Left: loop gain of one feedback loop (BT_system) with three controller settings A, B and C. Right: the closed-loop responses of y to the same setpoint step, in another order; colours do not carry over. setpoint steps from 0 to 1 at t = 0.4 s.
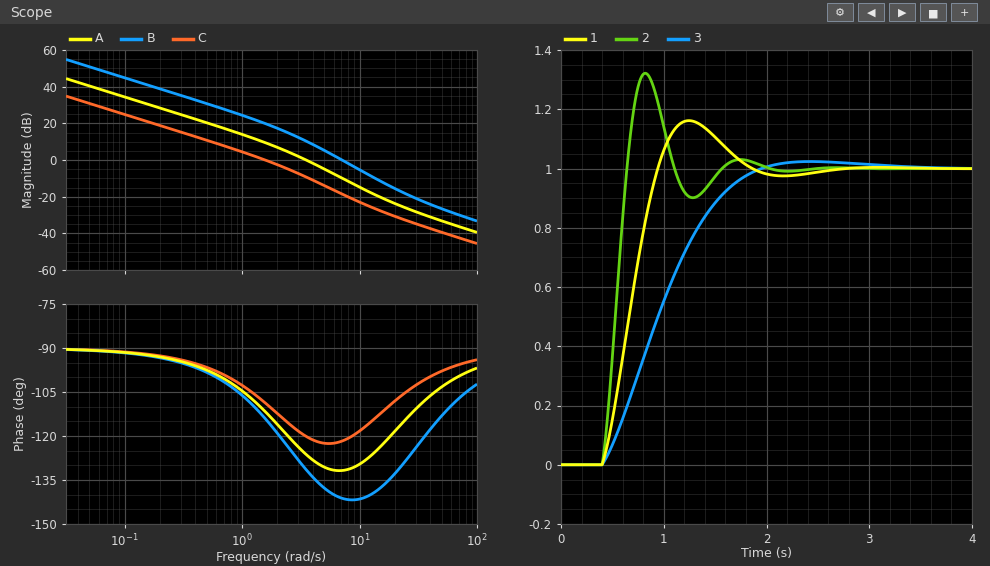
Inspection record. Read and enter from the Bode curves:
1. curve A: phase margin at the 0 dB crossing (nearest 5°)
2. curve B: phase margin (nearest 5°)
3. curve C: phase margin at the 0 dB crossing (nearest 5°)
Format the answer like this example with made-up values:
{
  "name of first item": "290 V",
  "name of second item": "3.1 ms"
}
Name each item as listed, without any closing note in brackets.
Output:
{
  "curve A: phase margin at the 0 dB crossing": "55°",
  "curve B: phase margin": "40°",
  "curve C: phase margin at the 0 dB crossing": "70°"
}
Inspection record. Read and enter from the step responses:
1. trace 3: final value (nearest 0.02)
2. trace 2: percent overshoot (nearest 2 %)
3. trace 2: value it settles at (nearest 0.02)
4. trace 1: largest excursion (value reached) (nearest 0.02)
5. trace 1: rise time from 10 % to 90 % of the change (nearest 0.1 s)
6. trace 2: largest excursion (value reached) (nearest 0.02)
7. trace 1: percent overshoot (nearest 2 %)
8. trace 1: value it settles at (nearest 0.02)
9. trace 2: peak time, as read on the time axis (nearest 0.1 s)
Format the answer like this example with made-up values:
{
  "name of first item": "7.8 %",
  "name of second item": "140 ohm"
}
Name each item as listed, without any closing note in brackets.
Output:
{
  "trace 3: final value": "1.00",
  "trace 2: percent overshoot": "32 %",
  "trace 2: value it settles at": "1.00",
  "trace 1: largest excursion (value reached)": "1.16",
  "trace 1: rise time from 10 % to 90 % of the change": "0.4 s",
  "trace 2: largest excursion (value reached)": "1.32",
  "trace 1: percent overshoot": "16 %",
  "trace 1: value it settles at": "1.00",
  "trace 2: peak time, as read on the time axis": "0.8 s"
}
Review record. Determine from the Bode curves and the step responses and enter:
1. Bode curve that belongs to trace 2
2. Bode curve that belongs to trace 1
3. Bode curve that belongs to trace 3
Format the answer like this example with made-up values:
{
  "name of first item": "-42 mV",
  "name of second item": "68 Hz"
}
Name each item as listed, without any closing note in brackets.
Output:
{
  "Bode curve that belongs to trace 2": "B",
  "Bode curve that belongs to trace 1": "A",
  "Bode curve that belongs to trace 3": "C"
}
